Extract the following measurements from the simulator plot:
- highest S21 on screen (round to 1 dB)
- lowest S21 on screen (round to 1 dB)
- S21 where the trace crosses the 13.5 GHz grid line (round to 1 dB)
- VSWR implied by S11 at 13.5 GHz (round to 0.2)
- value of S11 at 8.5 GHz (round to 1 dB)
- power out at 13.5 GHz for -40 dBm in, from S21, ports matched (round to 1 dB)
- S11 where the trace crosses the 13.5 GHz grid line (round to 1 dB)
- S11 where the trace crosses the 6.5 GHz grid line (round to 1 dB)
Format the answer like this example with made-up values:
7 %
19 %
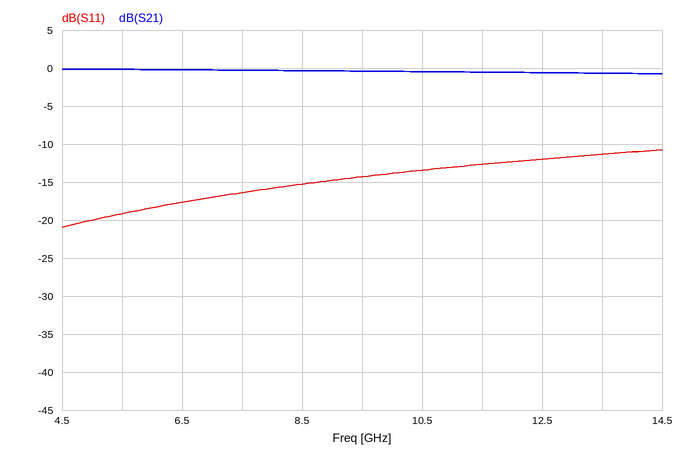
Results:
0 dB
-1 dB
-1 dB
1.8
-15 dB
-41 dBm
-11 dB
-18 dB
